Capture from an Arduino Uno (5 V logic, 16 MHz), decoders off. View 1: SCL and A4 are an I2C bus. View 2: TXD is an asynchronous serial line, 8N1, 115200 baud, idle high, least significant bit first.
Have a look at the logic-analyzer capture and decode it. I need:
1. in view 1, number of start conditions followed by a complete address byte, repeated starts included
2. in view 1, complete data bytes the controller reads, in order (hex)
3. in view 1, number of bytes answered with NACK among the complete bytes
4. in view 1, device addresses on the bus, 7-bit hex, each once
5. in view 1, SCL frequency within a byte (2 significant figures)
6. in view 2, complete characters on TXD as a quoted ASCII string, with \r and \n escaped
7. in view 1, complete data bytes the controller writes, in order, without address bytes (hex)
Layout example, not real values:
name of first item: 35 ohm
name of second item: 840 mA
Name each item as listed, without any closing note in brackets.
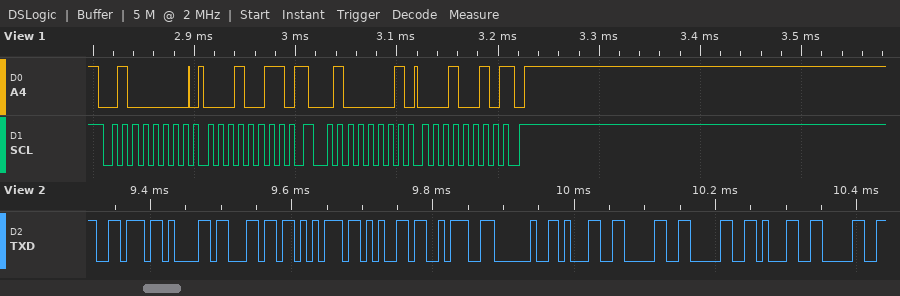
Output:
in view 1, number of start conditions followed by a complete address byte, repeated starts included: 2
in view 1, complete data bytes the controller reads, in order: 12
in view 1, number of bytes answered with NACK among the complete bytes: 1
in view 1, device addresses on the bus, 7-bit hex, each once: 0x20
in view 1, SCL frequency within a byte: 100 kHz
in view 2, complete characters on TXD as a quoted ASCII string, with \r and \n escaped: "value: 10010"
in view 1, complete data bytes the controller writes, in order, without address bytes: 13
